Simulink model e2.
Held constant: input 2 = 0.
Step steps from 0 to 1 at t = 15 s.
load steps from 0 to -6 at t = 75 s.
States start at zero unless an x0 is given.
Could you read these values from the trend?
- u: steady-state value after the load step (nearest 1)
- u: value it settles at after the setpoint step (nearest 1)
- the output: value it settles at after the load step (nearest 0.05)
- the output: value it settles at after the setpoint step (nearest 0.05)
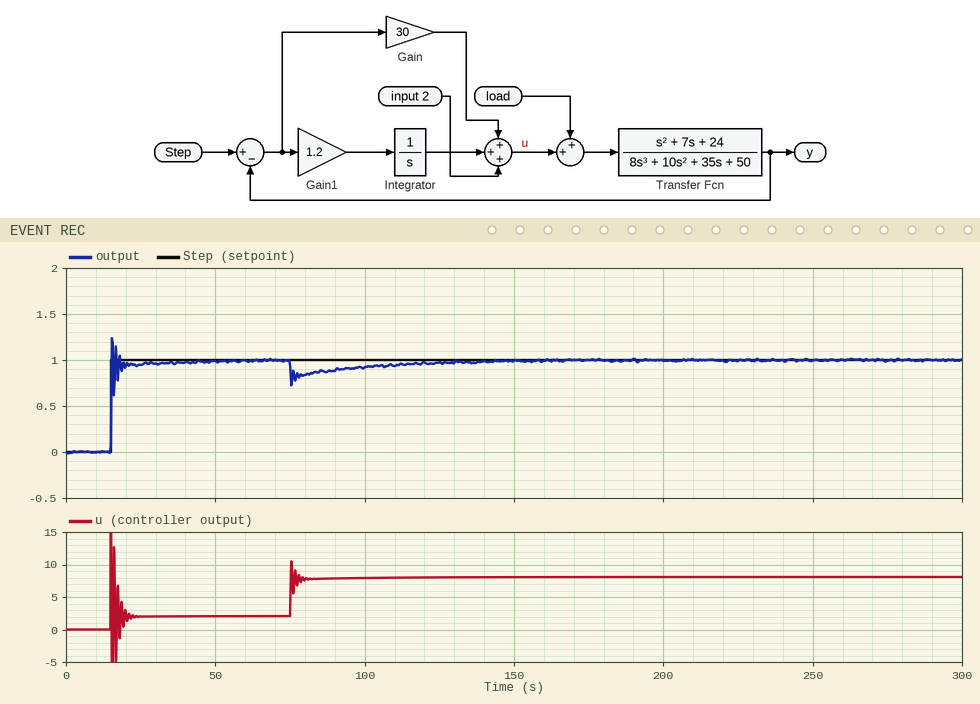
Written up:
8
2
1.00
1.00
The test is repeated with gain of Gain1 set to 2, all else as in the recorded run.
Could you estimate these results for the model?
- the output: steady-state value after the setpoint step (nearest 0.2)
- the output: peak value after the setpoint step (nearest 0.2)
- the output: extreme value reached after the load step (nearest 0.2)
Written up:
1.0
1.4
0.8
